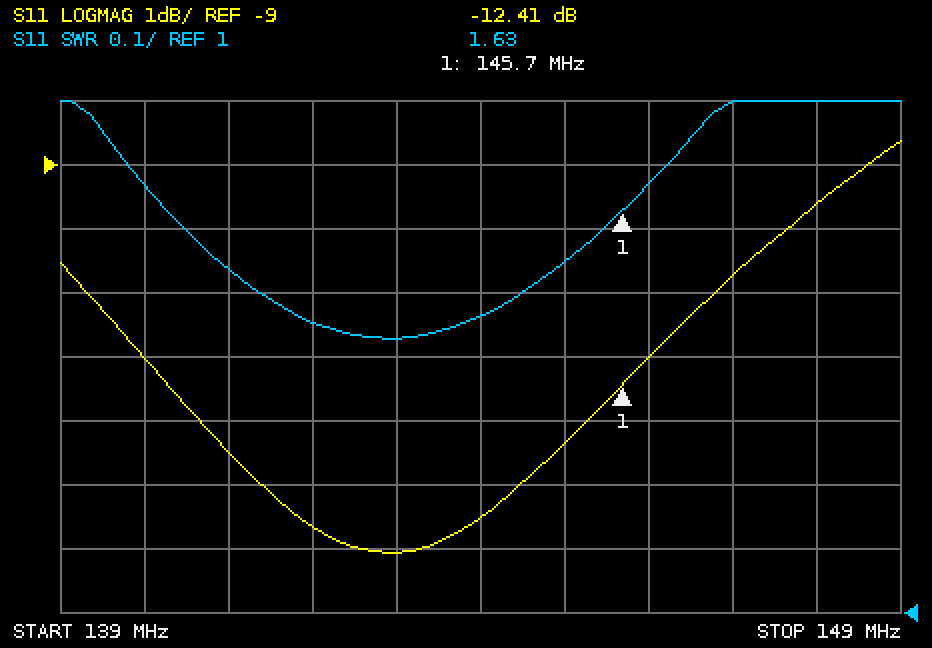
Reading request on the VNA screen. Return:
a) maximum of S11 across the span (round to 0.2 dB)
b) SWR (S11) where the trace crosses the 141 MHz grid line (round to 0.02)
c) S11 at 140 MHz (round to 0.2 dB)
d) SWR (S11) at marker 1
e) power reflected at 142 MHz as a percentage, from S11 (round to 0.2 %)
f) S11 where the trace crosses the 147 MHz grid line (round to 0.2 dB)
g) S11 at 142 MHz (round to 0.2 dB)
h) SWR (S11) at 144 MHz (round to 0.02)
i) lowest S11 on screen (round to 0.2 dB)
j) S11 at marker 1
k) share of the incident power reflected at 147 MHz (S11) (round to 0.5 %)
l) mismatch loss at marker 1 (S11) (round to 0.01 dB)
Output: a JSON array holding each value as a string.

["-8.6 dB", "1.54", "-12.0 dB", "1.63", "3.4 %", "-10.8 dB", "-14.6 dB", "1.46", "-15.0 dB", "-12.41 dB", "8.5 %", "0.26 dB"]
